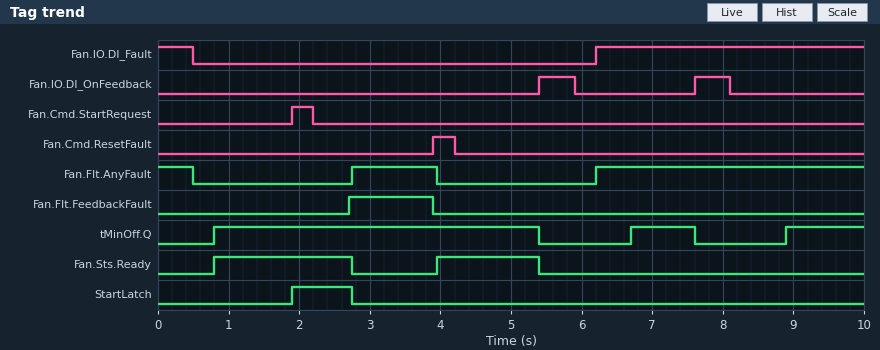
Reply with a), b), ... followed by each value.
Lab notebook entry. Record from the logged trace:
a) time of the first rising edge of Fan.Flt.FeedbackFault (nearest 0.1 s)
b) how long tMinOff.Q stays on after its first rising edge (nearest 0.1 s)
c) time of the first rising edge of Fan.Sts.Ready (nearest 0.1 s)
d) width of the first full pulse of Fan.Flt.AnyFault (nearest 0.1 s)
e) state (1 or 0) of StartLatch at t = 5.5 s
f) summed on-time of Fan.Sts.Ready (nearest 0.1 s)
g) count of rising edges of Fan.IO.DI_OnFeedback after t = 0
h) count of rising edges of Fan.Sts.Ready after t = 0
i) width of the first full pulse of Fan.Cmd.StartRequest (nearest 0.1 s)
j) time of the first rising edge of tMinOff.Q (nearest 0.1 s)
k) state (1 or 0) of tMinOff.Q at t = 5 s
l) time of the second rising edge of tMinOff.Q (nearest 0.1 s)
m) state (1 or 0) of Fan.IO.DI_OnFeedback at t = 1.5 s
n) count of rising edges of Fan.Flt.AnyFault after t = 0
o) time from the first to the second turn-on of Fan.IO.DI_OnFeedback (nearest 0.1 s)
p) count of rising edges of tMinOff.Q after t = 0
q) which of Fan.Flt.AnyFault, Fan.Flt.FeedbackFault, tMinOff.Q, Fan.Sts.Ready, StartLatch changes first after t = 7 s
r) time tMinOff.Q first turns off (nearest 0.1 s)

a) 2.7 s
b) 4.6 s
c) 0.8 s
d) 1.2 s
e) 0
f) 3.4 s
g) 2
h) 2
i) 0.3 s
j) 0.8 s
k) 1
l) 6.7 s
m) 0
n) 2
o) 2.2 s
p) 3
q) tMinOff.Q
r) 5.4 s
